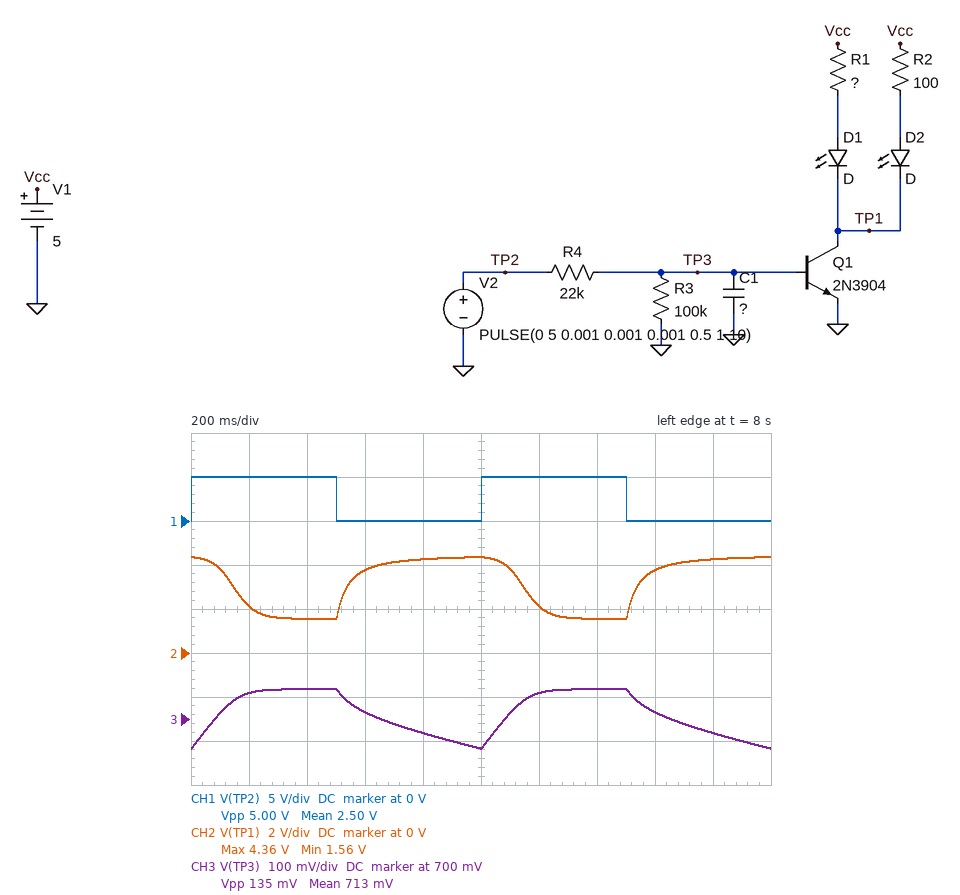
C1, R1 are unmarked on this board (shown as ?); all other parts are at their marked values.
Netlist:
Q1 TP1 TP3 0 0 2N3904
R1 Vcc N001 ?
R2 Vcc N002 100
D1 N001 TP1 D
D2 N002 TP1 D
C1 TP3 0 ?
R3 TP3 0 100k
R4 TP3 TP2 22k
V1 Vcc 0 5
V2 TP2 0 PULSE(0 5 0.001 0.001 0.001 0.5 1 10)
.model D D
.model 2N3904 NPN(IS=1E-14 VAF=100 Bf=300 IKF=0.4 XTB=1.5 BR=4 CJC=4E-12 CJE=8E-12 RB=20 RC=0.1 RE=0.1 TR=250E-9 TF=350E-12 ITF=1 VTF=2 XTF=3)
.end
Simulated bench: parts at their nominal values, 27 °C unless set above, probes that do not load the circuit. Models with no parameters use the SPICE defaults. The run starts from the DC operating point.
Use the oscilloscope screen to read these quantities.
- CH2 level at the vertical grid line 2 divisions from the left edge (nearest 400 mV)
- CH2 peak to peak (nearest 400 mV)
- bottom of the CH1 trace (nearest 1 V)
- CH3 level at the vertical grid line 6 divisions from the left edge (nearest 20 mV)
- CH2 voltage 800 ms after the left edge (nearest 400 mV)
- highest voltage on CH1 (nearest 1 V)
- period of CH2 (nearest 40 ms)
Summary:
1.6 V
2.8 V
0 V
760 mV
4.4 V
5 V
1.00 s
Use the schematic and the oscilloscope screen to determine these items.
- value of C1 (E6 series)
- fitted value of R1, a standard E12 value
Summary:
220 µF
120 Ω
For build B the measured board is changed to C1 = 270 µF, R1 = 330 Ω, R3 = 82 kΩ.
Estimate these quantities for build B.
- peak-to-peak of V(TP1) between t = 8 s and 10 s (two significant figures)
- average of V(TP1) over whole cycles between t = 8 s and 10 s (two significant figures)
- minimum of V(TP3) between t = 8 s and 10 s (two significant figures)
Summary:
3.8 V
2.8 V
650 mV
